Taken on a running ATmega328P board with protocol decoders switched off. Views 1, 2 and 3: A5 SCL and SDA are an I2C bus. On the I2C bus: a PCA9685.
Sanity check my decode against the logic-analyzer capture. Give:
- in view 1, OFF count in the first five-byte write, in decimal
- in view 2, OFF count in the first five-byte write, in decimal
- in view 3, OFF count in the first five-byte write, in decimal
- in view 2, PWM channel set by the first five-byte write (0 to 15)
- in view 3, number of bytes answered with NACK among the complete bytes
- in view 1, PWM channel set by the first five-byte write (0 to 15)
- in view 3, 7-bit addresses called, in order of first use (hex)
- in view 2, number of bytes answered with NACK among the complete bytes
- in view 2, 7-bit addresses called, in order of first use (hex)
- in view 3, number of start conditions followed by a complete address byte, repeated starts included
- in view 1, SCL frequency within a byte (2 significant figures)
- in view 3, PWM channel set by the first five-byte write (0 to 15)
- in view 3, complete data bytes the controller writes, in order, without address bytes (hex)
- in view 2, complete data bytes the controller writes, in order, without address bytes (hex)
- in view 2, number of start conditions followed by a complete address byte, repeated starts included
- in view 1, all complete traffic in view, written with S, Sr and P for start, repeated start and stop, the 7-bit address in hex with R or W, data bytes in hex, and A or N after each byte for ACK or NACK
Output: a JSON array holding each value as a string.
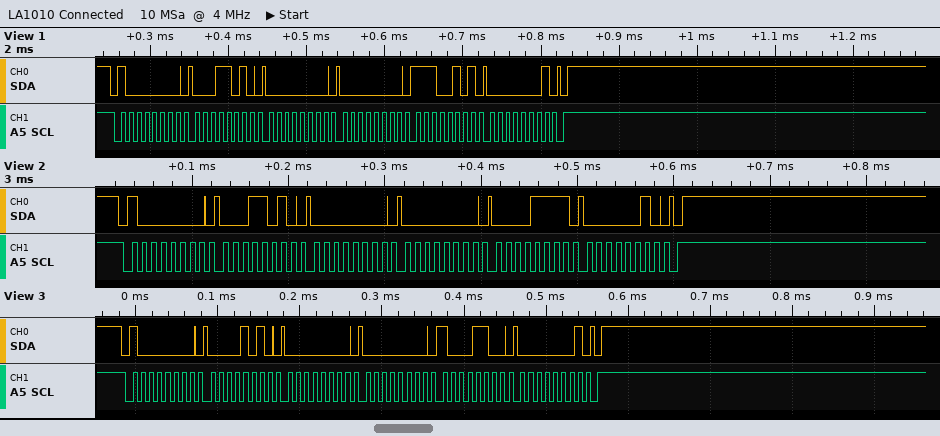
["485", "527", "396", "5", "0", "5", "0x40", "0", "0x40", "1", "100 kHz", "1", "0A 00 00 8C 01", "1A 00 00 0F 02", "1", "S 40W A 1A A 00 A 00 A E5 A 01 A P"]
